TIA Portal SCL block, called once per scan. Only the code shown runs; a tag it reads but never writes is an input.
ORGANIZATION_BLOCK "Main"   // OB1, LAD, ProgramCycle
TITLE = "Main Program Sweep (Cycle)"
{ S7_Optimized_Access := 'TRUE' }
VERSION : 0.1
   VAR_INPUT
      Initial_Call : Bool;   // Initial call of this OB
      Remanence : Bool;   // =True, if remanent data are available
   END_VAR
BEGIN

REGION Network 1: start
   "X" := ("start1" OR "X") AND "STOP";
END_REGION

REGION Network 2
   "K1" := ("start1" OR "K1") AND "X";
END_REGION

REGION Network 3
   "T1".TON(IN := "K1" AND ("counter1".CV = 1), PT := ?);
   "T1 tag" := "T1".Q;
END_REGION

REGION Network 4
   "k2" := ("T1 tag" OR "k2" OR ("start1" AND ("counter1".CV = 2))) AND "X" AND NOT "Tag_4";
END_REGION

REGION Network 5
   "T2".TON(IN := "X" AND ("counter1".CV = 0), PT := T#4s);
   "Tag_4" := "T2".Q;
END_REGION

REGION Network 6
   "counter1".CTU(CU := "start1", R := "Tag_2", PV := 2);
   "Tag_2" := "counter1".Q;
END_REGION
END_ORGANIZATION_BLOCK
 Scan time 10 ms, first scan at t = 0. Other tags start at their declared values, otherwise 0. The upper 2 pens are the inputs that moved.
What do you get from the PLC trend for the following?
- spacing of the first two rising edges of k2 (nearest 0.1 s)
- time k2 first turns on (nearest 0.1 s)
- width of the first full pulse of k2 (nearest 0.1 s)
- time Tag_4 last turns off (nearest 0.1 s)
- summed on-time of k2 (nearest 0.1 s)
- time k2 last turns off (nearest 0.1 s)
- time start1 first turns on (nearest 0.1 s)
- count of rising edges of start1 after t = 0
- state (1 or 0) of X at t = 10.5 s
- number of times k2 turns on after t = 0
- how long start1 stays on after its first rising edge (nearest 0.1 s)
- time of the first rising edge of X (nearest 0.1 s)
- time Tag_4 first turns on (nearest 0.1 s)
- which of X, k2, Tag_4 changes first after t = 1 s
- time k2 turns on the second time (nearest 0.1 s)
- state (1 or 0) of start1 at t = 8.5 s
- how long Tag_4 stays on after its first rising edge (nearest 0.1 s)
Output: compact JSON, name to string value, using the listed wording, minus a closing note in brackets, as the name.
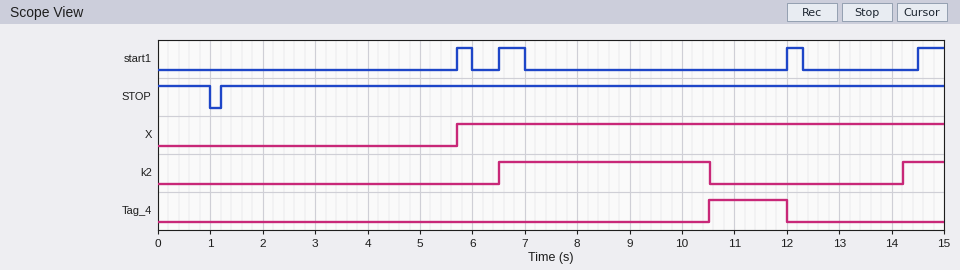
{"spacing of the first two rising edges of k2": "7.7 s", "time k2 first turns on": "6.5 s", "width of the first full pulse of k2": "4.0 s", "time Tag_4 last turns off": "12.0 s", "summed on-time of k2": "4.8 s", "time k2 last turns off": "10.5 s", "time start1 first turns on": "5.7 s", "count of rising edges of start1 after t = 0": "4", "state (1 or 0) of X at t = 10.5 s": "1", "number of times k2 turns on after t = 0": "2", "how long start1 stays on after its first rising edge": "0.3 s", "time of the first rising edge of X": "5.7 s", "time Tag_4 first turns on": "10.5 s", "which of X, k2, Tag_4 changes first after t = 1 s": "X", "time k2 turns on the second time": "14.2 s", "state (1 or 0) of start1 at t = 8.5 s": "0", "how long Tag_4 stays on after its first rising edge": "1.5 s"}
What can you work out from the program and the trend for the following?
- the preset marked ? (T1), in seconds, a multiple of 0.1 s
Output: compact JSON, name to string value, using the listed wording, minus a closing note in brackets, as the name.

{"the preset marked ? (T1), in seconds, a multiple of 0.1 s": "2.2 s"}
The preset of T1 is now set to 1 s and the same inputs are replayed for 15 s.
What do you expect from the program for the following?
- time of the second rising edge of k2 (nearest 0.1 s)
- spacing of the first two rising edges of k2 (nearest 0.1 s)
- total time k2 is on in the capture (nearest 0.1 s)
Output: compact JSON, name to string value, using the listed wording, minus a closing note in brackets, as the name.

{"time of the second rising edge of k2": "13.0 s", "spacing of the first two rising edges of k2": "6.5 s", "total time k2 is on in the capture": "6.0 s"}
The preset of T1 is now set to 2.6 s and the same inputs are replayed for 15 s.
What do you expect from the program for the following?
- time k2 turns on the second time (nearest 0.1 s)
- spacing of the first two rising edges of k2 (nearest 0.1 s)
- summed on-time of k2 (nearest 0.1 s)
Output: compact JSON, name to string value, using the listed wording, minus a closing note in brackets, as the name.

{"time k2 turns on the second time": "14.5 s", "spacing of the first two rising edges of k2": "8.0 s", "summed on-time of k2": "4.5 s"}
